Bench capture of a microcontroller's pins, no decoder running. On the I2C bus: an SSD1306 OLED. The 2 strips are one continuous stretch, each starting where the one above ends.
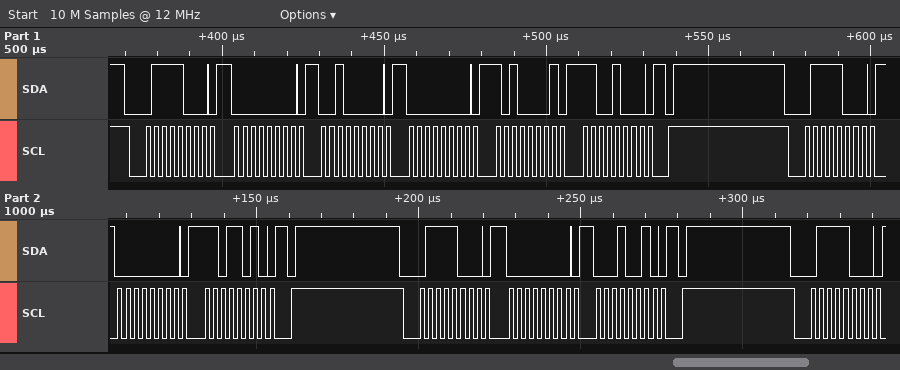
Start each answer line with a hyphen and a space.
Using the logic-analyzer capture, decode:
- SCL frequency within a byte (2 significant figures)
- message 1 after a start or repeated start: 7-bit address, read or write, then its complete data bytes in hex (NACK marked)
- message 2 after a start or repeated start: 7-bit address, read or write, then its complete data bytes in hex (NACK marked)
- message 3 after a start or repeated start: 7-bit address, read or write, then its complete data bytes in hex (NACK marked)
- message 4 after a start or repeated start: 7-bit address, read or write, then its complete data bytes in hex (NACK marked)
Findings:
- 400 kHz
- 0x3C write: 00 20 00 A1 C8
- 0x3C write: 00 DA
- 0x3C write: 00 12
- 0x3C write
